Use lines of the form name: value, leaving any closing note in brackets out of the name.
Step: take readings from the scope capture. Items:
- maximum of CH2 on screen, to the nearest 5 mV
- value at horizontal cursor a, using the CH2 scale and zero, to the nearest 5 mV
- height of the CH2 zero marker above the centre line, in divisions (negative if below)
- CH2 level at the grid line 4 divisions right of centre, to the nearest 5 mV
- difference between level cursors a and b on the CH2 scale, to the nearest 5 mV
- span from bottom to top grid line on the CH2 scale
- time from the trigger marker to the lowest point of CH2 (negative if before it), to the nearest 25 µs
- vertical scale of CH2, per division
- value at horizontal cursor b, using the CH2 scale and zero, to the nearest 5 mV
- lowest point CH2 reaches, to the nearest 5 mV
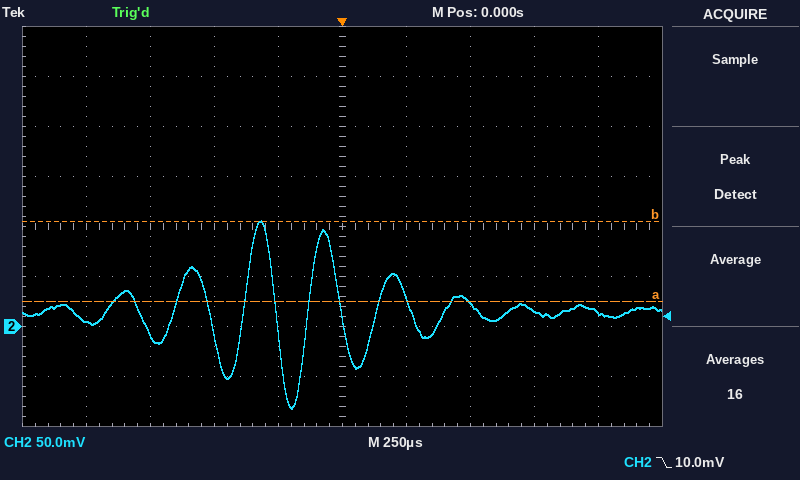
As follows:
maximum of CH2 on screen, to the nearest 5 mV: 105 mV
value at horizontal cursor a, using the CH2 scale and zero, to the nearest 5 mV: 25 mV
height of the CH2 zero marker above the centre line, in divisions: -2.0 div
CH2 level at the grid line 4 divisions right of centre, to the nearest 5 mV: 15 mV
difference between level cursors a and b on the CH2 scale, to the nearest 5 mV: 80 mV
span from bottom to top grid line on the CH2 scale: 400 mV
time from the trigger marker to the lowest point of CH2 (negative if before it), to the nearest 25 µs: -200 µs
vertical scale of CH2, per division: 50 mV
value at horizontal cursor b, using the CH2 scale and zero, to the nearest 5 mV: 105 mV
lowest point CH2 reaches, to the nearest 5 mV: -80 mV
